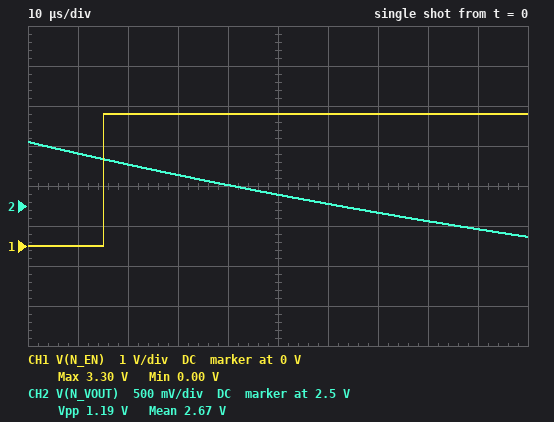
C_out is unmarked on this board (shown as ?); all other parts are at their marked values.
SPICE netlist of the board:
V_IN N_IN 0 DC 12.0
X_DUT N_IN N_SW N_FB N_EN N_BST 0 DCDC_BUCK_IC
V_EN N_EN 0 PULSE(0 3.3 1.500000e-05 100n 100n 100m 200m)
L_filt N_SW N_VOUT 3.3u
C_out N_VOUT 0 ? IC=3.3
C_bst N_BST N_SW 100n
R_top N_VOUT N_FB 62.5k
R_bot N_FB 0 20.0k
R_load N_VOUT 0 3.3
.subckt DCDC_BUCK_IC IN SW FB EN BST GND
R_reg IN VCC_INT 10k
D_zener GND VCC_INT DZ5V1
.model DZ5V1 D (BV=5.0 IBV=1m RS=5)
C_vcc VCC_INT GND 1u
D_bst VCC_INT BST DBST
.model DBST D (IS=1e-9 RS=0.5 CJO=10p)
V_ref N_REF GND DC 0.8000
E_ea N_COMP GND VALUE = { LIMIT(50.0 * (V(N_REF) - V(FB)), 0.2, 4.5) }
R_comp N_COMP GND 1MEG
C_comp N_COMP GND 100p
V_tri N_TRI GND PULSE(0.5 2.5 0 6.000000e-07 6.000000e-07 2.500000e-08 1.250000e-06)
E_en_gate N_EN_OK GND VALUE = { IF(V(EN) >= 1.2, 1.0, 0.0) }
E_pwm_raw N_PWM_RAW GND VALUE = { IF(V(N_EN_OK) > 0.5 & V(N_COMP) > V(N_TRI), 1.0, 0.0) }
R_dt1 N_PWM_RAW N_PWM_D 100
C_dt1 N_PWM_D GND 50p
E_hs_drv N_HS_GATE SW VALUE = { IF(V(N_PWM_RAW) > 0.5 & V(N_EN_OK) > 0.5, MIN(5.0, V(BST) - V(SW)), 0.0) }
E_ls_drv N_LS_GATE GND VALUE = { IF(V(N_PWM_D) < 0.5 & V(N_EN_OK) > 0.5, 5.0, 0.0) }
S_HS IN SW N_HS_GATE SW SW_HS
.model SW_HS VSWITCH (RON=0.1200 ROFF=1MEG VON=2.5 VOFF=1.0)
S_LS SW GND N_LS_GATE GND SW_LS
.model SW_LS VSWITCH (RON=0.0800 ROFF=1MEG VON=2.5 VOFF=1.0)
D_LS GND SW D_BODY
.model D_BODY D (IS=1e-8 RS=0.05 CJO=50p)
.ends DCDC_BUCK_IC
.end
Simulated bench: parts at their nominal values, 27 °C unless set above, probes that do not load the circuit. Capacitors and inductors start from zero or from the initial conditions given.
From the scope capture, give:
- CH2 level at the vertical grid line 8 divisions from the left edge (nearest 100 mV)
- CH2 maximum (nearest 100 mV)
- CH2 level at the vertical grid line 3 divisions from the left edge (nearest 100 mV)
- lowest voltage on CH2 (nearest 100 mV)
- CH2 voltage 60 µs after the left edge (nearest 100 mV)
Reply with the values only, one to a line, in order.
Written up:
2.3 V
3.3 V
2.9 V
2.1 V
2.5 V
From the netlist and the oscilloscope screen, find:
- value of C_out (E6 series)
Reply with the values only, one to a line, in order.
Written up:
68 µF
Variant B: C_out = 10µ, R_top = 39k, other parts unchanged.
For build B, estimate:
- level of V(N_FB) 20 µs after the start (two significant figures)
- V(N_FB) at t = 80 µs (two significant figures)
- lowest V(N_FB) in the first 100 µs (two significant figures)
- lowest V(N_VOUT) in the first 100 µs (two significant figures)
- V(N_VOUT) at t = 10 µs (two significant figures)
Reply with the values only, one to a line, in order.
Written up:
610 mV
99 mV
54 mV
160 mV
2.4 V
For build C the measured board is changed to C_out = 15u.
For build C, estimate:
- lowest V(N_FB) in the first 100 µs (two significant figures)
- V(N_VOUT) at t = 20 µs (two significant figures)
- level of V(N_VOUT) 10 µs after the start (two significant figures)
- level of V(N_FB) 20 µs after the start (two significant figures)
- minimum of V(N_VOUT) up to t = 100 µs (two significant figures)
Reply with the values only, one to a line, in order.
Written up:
110 mV
2.2 V
2.7 V
530 mV
440 mV
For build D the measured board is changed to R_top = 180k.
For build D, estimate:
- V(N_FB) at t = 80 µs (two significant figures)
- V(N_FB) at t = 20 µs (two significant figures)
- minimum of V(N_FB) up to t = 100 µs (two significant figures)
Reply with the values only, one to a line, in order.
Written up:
230 mV
300 mV
210 mV
